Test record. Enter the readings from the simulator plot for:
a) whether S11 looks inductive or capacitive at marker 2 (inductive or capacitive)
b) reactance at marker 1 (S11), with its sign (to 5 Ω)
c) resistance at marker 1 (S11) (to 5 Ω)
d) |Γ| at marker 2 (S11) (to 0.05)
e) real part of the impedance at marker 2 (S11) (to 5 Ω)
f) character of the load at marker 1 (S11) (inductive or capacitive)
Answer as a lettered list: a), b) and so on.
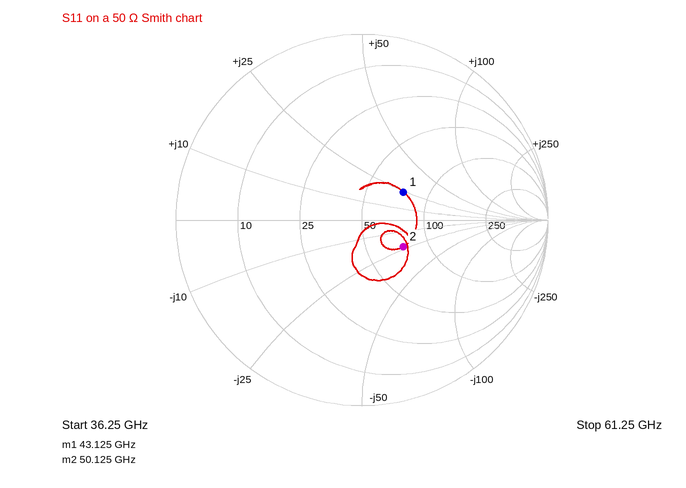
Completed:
a) capacitive
b) +25 Ω
c) 75 Ω
d) 0.25
e) 75 Ω
f) inductive
